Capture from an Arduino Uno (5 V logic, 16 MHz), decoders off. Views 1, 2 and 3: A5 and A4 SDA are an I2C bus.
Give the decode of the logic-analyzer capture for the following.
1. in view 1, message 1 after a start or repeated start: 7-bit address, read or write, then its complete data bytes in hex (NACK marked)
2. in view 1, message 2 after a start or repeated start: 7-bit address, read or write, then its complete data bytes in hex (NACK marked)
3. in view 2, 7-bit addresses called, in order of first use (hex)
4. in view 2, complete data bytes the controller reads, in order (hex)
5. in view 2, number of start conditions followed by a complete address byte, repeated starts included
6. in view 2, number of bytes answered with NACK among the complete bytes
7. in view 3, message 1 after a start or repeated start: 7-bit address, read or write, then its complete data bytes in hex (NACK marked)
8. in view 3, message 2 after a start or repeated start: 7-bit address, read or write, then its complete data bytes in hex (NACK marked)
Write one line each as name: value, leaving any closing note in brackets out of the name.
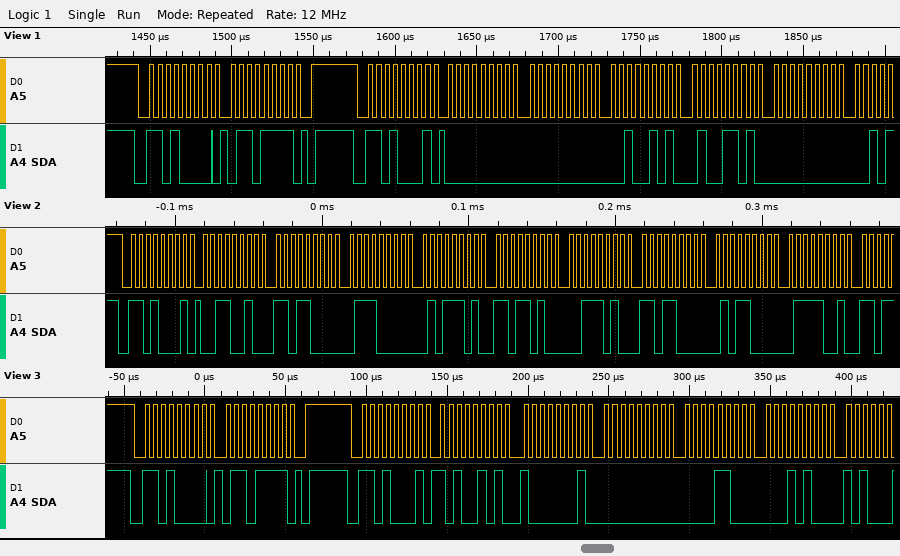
in view 1, message 1 after a start or repeated start: 7-bit address, read or write, then its complete data bytes in hex: 0x68 write: 6F
in view 1, message 2 after a start or repeated start: 7-bit address, read or write, then its complete data bytes in hex: 0x68 read: 00 00 25 4D 00
in view 2, 7-bit addresses called, in order of first use: 0x68
in view 2, complete data bytes the controller reads, in order: 32 D8 70 5D DA 3A D8 58 79
in view 2, number of start conditions followed by a complete address byte, repeated starts included: 1
in view 2, number of bytes answered with NACK among the complete bytes: 0
in view 3, message 1 after a start or repeated start: 7-bit address, read or write, then its complete data bytes in hex: 0x68 write: 6F
in view 3, message 2 after a start or repeated start: 7-bit address, read or write, then its complete data bytes in hex: 0x68 read: A5 81 00 0C 14
